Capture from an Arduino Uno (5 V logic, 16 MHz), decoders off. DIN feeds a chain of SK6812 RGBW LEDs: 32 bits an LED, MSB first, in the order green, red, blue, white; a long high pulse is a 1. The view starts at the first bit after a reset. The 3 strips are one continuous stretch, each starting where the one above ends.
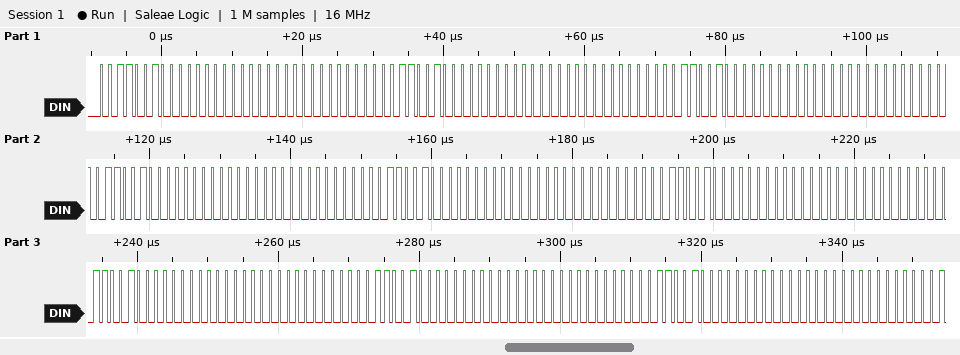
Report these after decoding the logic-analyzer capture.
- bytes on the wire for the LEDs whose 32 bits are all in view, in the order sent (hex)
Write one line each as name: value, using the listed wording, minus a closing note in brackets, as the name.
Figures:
bytes on the wire for the LEDs whose 32 bits are all in view, in the order sent: 32 00 00 00 32 00 00 00 32 00 00 00 32 00 00 00 32 00 00 00 32 00 00 00 32 00 00 00 32 00 00 00 32 00 00 00
